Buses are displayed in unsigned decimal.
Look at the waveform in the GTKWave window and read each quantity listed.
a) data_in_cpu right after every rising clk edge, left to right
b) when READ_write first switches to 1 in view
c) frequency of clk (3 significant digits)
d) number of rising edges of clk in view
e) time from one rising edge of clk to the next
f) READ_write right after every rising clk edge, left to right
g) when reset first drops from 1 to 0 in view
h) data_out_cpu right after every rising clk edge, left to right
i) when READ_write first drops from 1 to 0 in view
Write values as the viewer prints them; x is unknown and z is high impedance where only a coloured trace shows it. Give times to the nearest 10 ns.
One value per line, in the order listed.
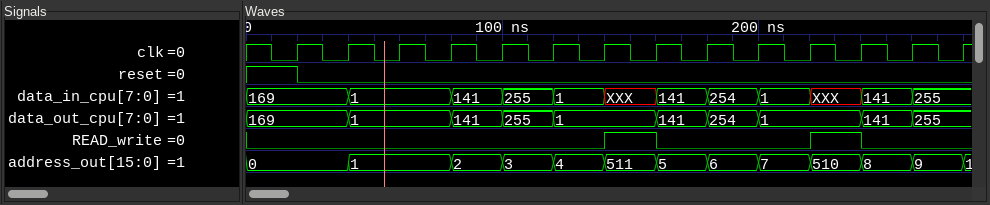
169, 1, 1, 141, 255, 1, XXX, 141, 254, 1, XXX, 141, 255, 255
140 ns
50.0 MHz
14
20 ns
0 0 0 0 0 0 1 0 0 0 1 0 0 0
20 ns
169, 1, 1, 141, 255, 1, 1, 141, 254, 1, 1, 141, 255, 255
160 ns
